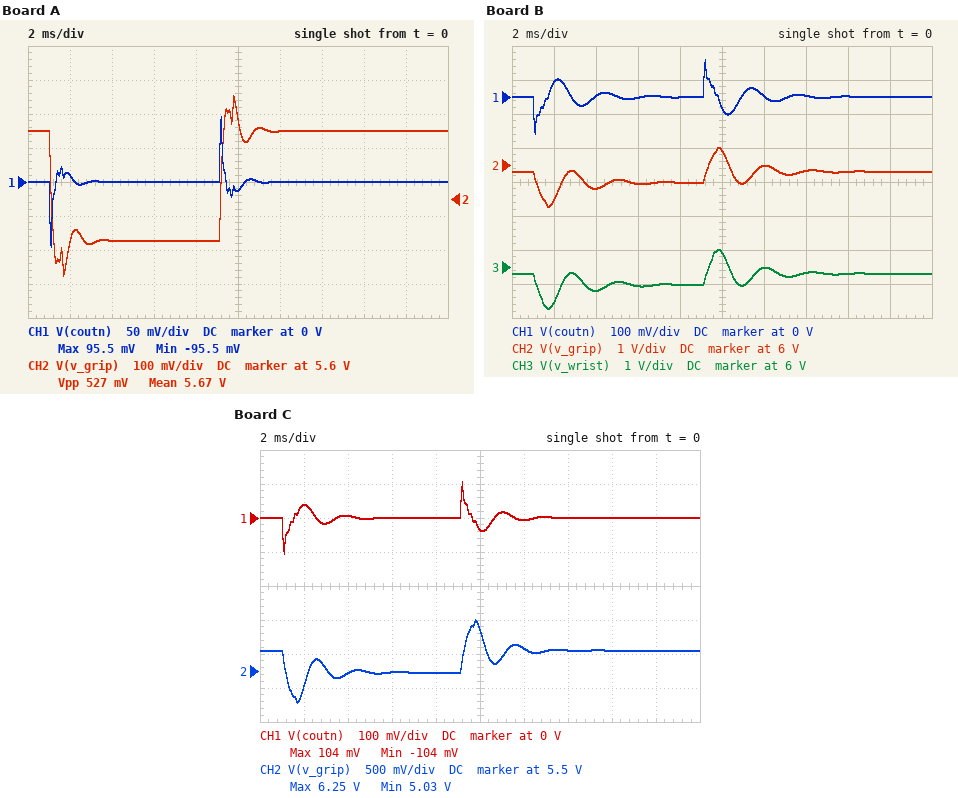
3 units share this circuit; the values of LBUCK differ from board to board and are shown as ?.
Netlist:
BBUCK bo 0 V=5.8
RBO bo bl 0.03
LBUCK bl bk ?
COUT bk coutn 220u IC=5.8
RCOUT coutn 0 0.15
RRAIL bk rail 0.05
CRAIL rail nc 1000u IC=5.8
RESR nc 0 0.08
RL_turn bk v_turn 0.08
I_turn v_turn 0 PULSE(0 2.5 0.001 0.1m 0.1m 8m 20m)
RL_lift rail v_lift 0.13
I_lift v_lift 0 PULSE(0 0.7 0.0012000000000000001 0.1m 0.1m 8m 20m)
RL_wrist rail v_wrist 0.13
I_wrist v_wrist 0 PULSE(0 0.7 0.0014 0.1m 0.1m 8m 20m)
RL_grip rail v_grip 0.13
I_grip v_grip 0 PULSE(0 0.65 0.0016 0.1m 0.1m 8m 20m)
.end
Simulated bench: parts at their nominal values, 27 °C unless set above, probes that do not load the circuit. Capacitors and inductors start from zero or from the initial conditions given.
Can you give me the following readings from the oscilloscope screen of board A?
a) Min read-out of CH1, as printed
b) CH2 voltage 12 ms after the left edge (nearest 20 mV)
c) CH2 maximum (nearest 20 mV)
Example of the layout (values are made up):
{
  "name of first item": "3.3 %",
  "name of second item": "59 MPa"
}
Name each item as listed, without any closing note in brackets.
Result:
{
  "Min read-out of CH1, as printed": "-95.5 mV",
  "CH2 voltage 12 ms after the left edge": "5.80 V",
  "CH2 maximum": "5.90 V"
}
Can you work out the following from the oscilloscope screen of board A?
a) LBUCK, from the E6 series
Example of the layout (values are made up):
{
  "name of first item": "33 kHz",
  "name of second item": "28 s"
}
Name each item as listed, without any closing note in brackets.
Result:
{
  "LBUCK, from the E6 series": "33 µH"
}
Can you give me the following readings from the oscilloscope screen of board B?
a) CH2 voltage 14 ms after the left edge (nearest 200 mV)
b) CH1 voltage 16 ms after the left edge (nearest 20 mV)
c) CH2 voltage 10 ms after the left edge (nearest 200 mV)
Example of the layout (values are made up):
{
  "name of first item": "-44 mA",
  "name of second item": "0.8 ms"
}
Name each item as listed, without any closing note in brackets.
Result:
{
  "CH2 voltage 14 ms after the left edge": "5.8 V",
  "CH1 voltage 16 ms after the left edge": "0 V",
  "CH2 voltage 10 ms after the left edge": "6.4 V"
}
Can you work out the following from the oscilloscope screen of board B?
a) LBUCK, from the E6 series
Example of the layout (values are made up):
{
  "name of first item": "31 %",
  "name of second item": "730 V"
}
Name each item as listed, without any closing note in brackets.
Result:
{
  "LBUCK, from the E6 series": "100 µH"
}
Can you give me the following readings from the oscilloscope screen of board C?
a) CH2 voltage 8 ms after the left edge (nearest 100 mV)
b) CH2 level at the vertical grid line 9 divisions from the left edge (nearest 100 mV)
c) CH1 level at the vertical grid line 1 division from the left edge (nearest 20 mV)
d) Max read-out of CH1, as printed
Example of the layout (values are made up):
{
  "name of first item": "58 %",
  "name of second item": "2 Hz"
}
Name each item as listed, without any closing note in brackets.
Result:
{
  "CH2 voltage 8 ms after the left edge": "5.5 V",
  "CH2 level at the vertical grid line 9 divisions from the left edge": "5.8 V",
  "CH1 level at the vertical grid line 1 division from the left edge": "40 mV",
  "Max read-out of CH1, as printed": "104 mV"
}
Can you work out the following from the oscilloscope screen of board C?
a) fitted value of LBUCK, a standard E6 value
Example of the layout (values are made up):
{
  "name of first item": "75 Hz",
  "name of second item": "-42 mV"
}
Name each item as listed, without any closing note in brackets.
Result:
{
  "fitted value of LBUCK, a standard E6 value": "68 µH"
}
